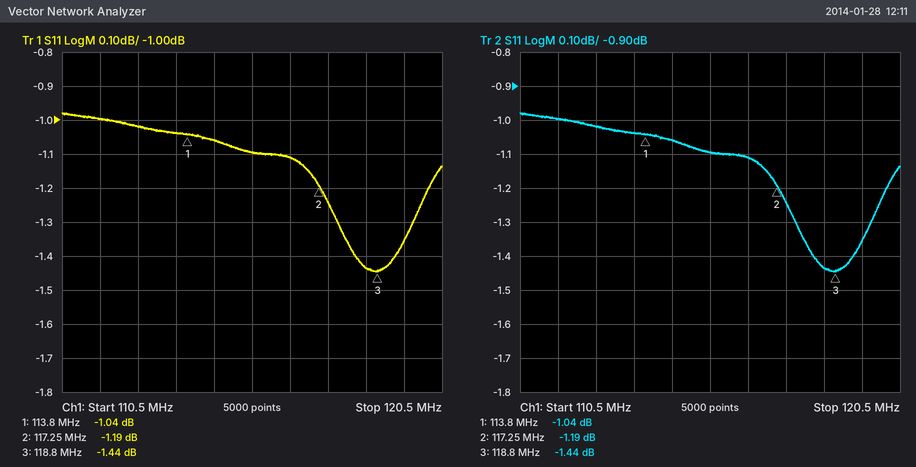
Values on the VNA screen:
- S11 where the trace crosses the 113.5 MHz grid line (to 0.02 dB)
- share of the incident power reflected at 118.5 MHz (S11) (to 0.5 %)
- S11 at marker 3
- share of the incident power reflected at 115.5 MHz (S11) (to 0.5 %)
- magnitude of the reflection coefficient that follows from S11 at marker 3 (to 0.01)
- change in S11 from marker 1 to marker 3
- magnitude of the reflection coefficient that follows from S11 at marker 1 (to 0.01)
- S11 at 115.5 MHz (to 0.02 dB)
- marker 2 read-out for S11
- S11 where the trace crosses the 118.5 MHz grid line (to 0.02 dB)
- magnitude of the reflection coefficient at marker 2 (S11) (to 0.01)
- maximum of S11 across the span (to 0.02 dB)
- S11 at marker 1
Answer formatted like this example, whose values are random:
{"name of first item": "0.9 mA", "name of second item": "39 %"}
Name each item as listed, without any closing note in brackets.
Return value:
{"S11 where the trace crosses the 113.5 MHz grid line": "-1.04 dB", "share of the incident power reflected at 118.5 MHz (S11)": "72.0 %", "S11 at marker 3": "-1.44 dB", "share of the incident power reflected at 115.5 MHz (S11)": "77.5 %", "magnitude of the reflection coefficient that follows from S11 at marker 3": "0.85", "change in S11 from marker 1 to marker 3": "-0.40 dB", "magnitude of the reflection coefficient that follows from S11 at marker 1": "0.89", "S11 at 115.5 MHz": "-1.10 dB", "marker 2 read-out for S11": "-1.19 dB", "S11 where the trace crosses the 118.5 MHz grid line": "-1.44 dB", "magnitude of the reflection coefficient at marker 2 (S11)": "0.87", "maximum of S11 across the span": "-0.98 dB", "S11 at marker 1": "-1.04 dB"}
